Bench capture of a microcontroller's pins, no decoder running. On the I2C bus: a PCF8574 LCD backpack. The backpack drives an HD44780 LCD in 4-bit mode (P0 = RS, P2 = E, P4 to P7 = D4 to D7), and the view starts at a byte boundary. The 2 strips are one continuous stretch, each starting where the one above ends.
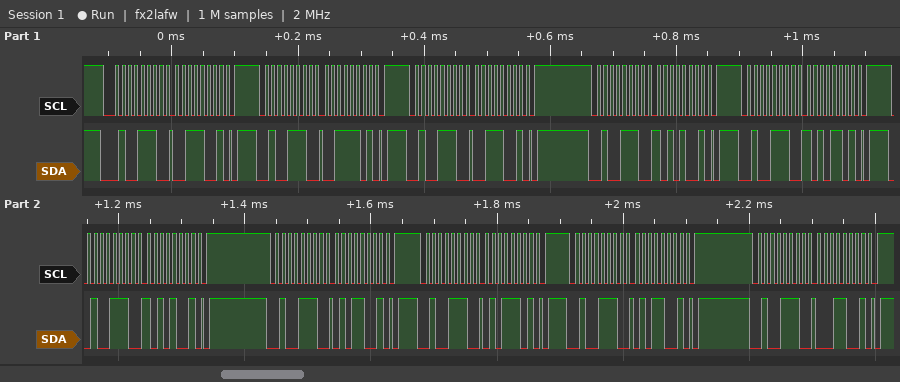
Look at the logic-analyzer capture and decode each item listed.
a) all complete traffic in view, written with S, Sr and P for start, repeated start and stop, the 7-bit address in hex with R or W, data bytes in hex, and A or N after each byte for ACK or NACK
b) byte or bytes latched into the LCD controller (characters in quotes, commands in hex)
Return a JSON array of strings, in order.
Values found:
["S 27W A 39 A P S 27W A 3D A P S 27W A 39 A P S 27W A A9 A P S 27W A AD A P S 27W A A9 A P S 27W A 59 A P S 27W A 5D A P S 27W A 59 A P S 27W A 19 A P", "':'"]
